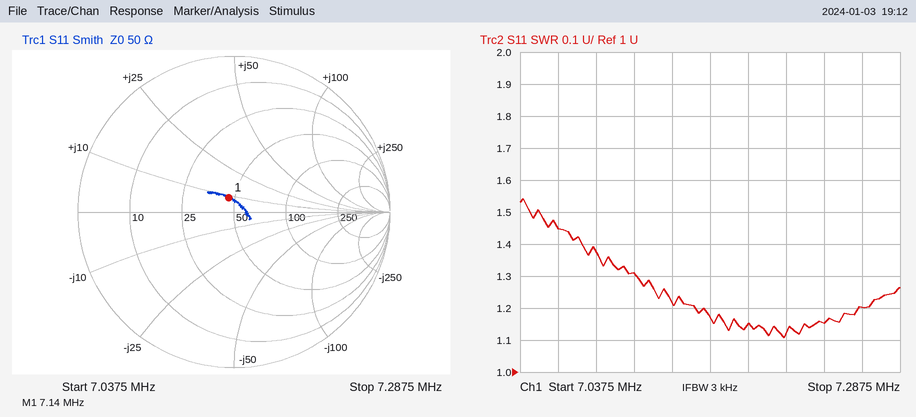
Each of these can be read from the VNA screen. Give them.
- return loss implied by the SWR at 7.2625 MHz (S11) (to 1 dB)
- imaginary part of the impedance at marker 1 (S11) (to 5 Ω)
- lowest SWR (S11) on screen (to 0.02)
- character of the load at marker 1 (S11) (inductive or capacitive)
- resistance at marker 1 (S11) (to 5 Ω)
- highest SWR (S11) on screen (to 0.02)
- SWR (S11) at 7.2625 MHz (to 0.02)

21 dB
+10 Ω
1.10
inductive
45 Ω
1.54
1.20
